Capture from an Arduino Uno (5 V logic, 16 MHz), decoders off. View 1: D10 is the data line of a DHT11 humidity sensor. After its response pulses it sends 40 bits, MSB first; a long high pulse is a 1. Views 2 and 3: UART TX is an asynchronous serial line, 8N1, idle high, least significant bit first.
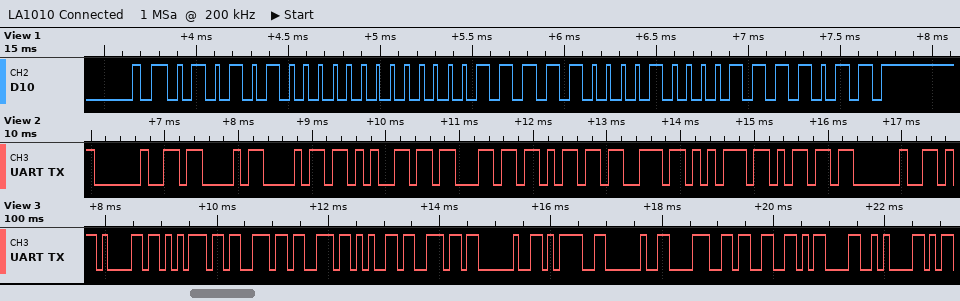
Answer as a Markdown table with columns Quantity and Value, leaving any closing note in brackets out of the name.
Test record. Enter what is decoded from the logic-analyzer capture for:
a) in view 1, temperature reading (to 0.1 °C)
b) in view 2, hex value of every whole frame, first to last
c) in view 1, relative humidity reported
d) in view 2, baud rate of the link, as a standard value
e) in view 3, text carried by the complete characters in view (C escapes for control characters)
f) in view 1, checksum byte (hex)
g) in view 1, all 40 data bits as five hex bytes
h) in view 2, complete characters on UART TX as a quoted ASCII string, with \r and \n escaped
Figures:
| Quantity | Value |
|---|---|
| in view 1, temperature reading | 31.8 °C |
| in view 2, hex value of every whole frame, first to last | 0x20 0x43 0x68 0x65 0x63 0x6B 0x73 0x75 0x6D 0x20 |
| in view 1, relative humidity reported | 84 % |
| in view 2, baud rate of the link, as a standard value | 9600 baud |
| in view 3, text carried by the complete characters in view | "aussen = 83\r\n" |
| in view 1, checksum byte | 0x7B |
| in view 1, all 40 data bits as five hex bytes | 54 00 1F 08 7B |
| in view 2, complete characters on UART TX as a quoted ASCII string, with \r and \n escaped | " Checksum " |
